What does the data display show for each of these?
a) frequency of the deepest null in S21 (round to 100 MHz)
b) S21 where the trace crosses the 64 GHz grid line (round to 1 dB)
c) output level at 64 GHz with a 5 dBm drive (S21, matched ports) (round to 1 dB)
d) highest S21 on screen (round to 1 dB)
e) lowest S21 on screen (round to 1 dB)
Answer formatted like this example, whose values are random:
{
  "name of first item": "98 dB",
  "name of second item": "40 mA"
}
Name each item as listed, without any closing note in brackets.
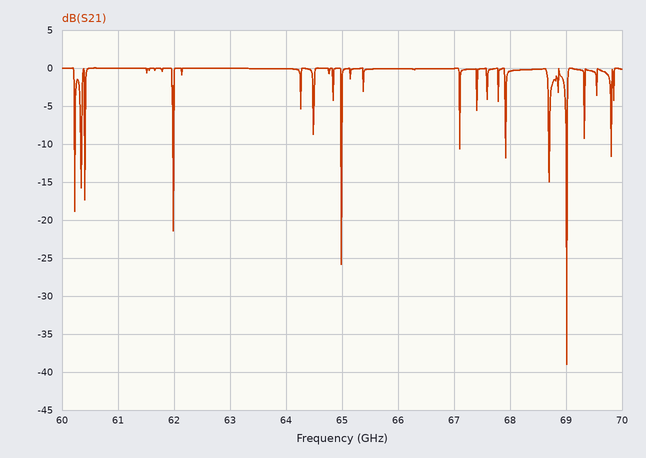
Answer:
{
  "frequency of the deepest null in S21": "69.0 GHz",
  "S21 where the trace crosses the 64 GHz grid line": "0 dB",
  "output level at 64 GHz with a 5 dBm drive (S21, matched ports)": "5 dBm",
  "highest S21 on screen": "0 dB",
  "lowest S21 on screen": "-39 dB"
}
